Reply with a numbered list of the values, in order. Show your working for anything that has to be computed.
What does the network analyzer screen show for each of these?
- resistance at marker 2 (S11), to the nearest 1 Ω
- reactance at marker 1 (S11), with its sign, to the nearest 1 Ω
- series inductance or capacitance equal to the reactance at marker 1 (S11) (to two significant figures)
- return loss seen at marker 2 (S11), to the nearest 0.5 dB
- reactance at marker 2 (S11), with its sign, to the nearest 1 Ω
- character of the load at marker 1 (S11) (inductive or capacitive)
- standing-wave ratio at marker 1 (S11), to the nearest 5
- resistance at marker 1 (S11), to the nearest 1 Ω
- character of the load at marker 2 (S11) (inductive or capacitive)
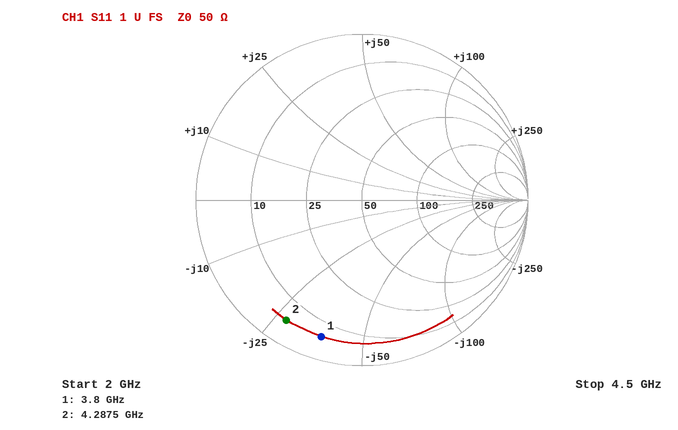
1. 5 Ω
2. -37 Ω
3. C = 1/(2π × 3.8 GHz × 37 Ω) ≈ 1.1 pF
4. 1.5 dB
5. -27 Ω
6. capacitive
7. 15
8. 6 Ω
9. capacitive
